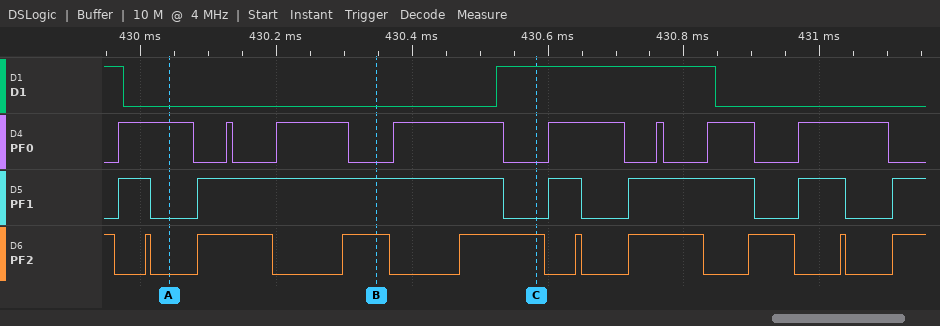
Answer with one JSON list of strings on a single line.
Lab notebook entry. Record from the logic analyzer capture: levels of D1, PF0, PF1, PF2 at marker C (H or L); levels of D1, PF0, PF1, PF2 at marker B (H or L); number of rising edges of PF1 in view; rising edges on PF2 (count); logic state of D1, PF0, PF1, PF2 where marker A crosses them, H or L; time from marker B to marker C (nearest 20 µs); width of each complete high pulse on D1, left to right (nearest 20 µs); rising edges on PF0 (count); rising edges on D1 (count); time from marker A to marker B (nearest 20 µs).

["D1=H, PF0=L, PF1=L, PF2=H", "D1=L, PF0=L, PF1=H, PF2=H", "6", "9", "D1=L, PF0=H, PF1=L, PF2=L", "240 µs", "320 µs", "8", "1", "300 µs"]
